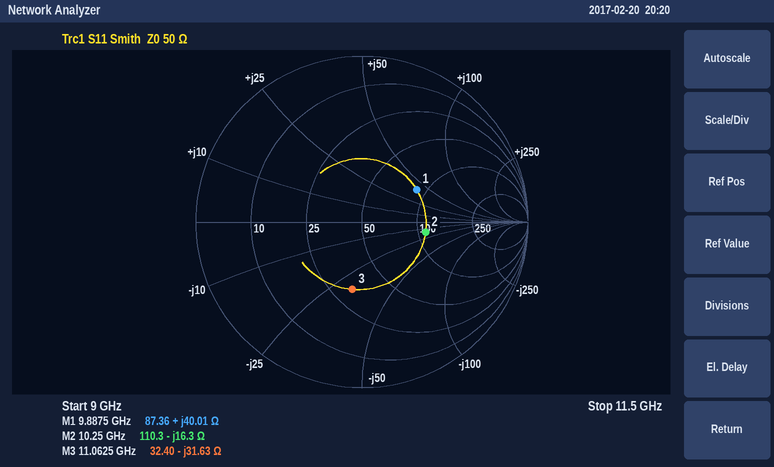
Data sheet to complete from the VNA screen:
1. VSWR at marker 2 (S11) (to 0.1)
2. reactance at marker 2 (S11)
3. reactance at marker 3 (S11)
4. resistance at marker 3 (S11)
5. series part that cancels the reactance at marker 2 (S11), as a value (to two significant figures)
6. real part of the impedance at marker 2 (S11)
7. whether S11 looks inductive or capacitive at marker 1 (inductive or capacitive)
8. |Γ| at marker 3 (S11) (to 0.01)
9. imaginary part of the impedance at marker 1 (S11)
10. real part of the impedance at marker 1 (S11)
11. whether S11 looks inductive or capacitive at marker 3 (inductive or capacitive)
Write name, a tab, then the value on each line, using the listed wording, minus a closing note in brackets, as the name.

VSWR at marker 2 (S11)	2.3
reactance at marker 2	-16.3 Ω
reactance at marker 3	-31.63 Ω
resistance at marker 3	32.40 Ω
series part that cancels the reactance at marker 2 (S11), as a value	250 pH
real part of the impedance at marker 2	110.3 Ω
whether S11 looks inductive or capacitive at marker 1	inductive
|Γ| at marker 3 (S11)	0.41
imaginary part of the impedance at marker 1	+40.01 Ω
real part of the impedance at marker 1	87.36 Ω
whether S11 looks inductive or capacitive at marker 3	capacitive
